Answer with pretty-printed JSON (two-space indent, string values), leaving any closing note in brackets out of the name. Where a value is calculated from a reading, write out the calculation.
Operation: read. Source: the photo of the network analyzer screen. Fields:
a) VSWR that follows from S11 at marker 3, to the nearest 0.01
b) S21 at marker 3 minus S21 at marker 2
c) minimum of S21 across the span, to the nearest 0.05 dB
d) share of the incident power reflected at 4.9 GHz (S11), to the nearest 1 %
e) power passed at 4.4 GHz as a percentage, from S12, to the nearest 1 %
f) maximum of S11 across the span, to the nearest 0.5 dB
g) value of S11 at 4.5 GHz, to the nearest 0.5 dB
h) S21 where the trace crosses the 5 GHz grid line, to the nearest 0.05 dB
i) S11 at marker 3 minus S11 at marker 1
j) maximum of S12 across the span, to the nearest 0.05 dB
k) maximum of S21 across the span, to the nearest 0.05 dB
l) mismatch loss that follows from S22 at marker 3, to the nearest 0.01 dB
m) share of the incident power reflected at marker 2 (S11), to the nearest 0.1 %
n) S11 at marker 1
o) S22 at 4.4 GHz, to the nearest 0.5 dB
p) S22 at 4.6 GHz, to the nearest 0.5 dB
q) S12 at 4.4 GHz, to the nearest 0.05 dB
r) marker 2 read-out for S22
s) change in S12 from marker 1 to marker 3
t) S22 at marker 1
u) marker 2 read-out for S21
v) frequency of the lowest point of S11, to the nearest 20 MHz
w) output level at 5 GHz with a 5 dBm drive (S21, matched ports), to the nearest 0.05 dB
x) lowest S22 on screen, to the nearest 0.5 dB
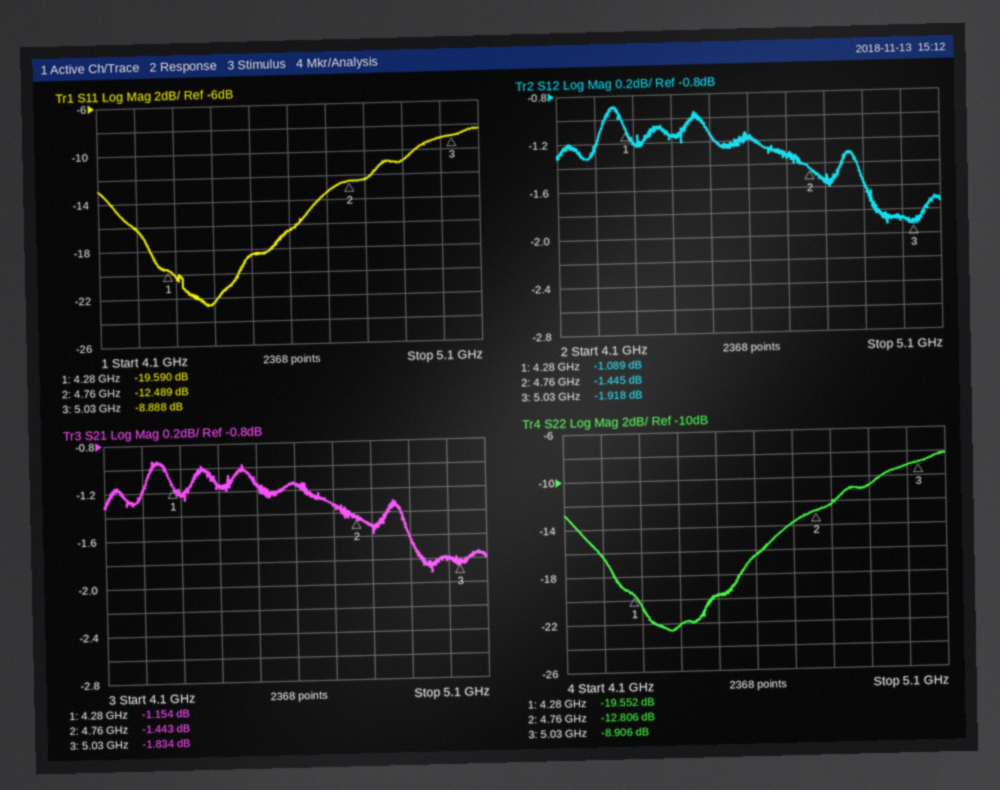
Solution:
{
  "VSWR that follows from S11 at marker 3, to the nearest 0.01": "(1 + 0.3594)/(1 − 0.3594) ≈ 2.12",
  "S21 at marker 3 minus S21 at marker 2": "-1.834 − (-1.443) = -0.391 dB",
  "minimum of S21 across the span, to the nearest 0.05 dB": "-1.90 dB",
  "share of the incident power reflected at 4.9 GHz (S11), to the nearest 1 %": "10^(-11/10) ≈ 8 %",
  "power passed at 4.4 GHz as a percentage, from S12, to the nearest 1 %": "10^(-1.15/10) ≈ 77 %",
  "maximum of S11 across the span, to the nearest 0.5 dB": "-8.5 dB",
  "value of S11 at 4.5 GHz, to the nearest 0.5 dB": "-18.5 dB",
  "S21 where the trace crosses the 5 GHz grid line, to the nearest 0.05 dB": "-1.80 dB",
  "S11 at marker 3 minus S11 at marker 1": "-8.888 − (-19.59) = 10.702 dB",
  "maximum of S12 across the span, to the nearest 0.05 dB": "-0.90 dB",
  "maximum of S21 across the span, to the nearest 0.05 dB": "-0.95 dB",
  "mismatch loss that follows from S22 at marker 3, to the nearest 0.01 dB": "−10 log10(1 − 10^(-8.906/10)) ≈ 0.60 dB",
  "share of the incident power reflected at marker 2 (S11), to the nearest 0.1 %": "10^(-12.489/10) ≈ 5.6 %",
  "S11 at marker 1": "-19.590 dB",
  "S22 at 4.4 GHz, to the nearest 0.5 dB": "-22.0 dB",
  "S22 at 4.6 GHz, to the nearest 0.5 dB": "-16.5 dB",
  "S12 at 4.4 GHz, to the nearest 0.05 dB": "-1.15 dB",
  "marker 2 read-out for S22": "-12.806 dB",
  "change in S12 from marker 1 to marker 3": "-1.918 − (-1.089) = -0.829 dB",
  "S22 at marker 1": "-19.552 dB",
  "marker 2 read-out for S21": "-1.443 dB",
  "frequency of the lowest point of S11, to the nearest 20 MHz": "4.38 GHz",
  "output level at 5 GHz with a 5 dBm drive (S21, matched ports), to the nearest 0.05 dB": "5 dBm + (-1.80 dB) = 3.20 dBm",
  "lowest S22 on screen, to the nearest 0.5 dB": "-22.5 dB"
}
